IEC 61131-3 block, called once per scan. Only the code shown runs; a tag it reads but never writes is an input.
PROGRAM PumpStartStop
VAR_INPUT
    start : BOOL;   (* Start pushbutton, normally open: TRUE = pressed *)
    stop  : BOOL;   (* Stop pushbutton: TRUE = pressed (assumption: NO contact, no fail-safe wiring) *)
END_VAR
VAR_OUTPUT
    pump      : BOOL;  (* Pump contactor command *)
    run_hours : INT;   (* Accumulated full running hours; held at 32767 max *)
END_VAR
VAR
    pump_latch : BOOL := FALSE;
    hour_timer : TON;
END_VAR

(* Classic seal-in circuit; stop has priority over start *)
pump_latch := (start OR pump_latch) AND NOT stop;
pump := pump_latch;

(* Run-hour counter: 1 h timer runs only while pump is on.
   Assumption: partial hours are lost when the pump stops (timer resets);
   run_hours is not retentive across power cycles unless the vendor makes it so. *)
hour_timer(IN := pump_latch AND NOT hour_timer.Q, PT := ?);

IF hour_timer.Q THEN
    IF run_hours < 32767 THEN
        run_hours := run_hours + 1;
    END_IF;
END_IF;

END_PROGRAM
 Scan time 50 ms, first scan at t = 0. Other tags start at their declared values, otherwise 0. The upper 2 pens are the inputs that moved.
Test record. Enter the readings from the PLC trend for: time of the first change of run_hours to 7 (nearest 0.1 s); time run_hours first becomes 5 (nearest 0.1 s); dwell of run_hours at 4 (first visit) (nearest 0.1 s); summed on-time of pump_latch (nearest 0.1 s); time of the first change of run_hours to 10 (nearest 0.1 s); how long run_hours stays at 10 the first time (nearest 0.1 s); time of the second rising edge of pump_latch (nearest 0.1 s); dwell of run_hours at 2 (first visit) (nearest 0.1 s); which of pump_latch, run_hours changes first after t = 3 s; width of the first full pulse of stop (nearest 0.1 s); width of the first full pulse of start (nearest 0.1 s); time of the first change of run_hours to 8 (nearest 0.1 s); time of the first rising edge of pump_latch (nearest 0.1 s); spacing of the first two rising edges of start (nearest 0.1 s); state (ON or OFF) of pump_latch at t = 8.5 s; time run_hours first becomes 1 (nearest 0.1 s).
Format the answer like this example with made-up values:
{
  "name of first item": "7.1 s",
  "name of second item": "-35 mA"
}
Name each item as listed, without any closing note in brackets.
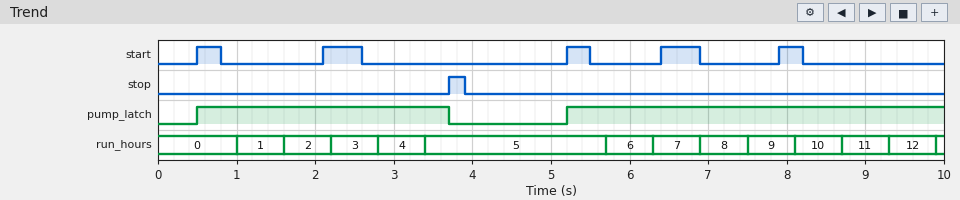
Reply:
{
  "time of the first change of run_hours to 7": "6.3 s",
  "time run_hours first becomes 5": "3.4 s",
  "dwell of run_hours at 4 (first visit)": "0.6 s",
  "summed on-time of pump_latch": "8.0 s",
  "time of the first change of run_hours to 10": "8.1 s",
  "how long run_hours stays at 10 the first time": "0.6 s",
  "time of the second rising edge of pump_latch": "5.2 s",
  "dwell of run_hours at 2 (first visit)": "0.6 s",
  "which of pump_latch, run_hours changes first after t = 3 s": "run_hours",
  "width of the first full pulse of stop": "0.2 s",
  "width of the first full pulse of start": "0.3 s",
  "time of the first change of run_hours to 8": "6.9 s",
  "time of the first rising edge of pump_latch": "0.5 s",
  "spacing of the first two rising edges of start": "1.6 s",
  "state (ON or OFF) of pump_latch at t = 8.5 s": "ON",
  "time run_hours first becomes 1": "1.0 s"
}
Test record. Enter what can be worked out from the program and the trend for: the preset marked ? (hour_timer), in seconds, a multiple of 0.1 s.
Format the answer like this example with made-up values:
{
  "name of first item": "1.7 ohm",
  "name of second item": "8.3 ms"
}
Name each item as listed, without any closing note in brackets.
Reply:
{
  "the preset marked ? (hour_timer), in seconds, a multiple of 0.1 s": "0.5 s"
}
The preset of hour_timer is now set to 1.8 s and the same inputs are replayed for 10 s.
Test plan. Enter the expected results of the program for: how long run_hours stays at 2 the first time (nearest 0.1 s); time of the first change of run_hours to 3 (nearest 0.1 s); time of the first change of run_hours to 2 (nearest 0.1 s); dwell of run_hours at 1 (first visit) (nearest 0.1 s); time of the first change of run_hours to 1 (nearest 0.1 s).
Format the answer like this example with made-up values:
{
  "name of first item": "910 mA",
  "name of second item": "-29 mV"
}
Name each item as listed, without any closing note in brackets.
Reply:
{
  "how long run_hours stays at 2 the first time": "1.9 s",
  "time of the first change of run_hours to 3": "8.9 s",
  "time of the first change of run_hours to 2": "7.0 s",
  "dwell of run_hours at 1 (first visit)": "4.7 s",
  "time of the first change of run_hours to 1": "2.3 s"
}
